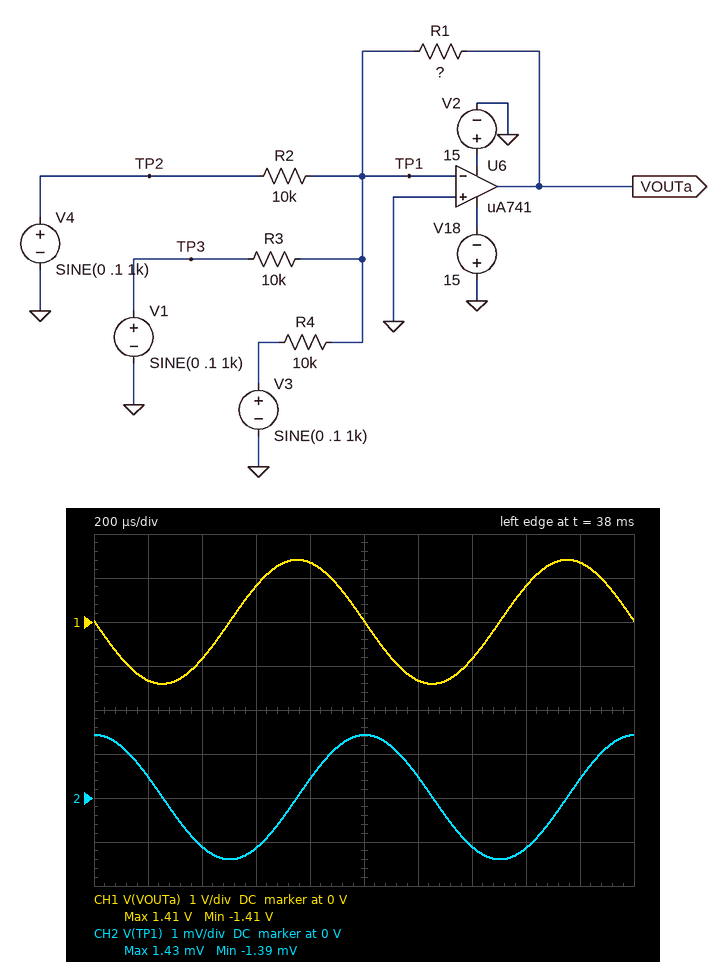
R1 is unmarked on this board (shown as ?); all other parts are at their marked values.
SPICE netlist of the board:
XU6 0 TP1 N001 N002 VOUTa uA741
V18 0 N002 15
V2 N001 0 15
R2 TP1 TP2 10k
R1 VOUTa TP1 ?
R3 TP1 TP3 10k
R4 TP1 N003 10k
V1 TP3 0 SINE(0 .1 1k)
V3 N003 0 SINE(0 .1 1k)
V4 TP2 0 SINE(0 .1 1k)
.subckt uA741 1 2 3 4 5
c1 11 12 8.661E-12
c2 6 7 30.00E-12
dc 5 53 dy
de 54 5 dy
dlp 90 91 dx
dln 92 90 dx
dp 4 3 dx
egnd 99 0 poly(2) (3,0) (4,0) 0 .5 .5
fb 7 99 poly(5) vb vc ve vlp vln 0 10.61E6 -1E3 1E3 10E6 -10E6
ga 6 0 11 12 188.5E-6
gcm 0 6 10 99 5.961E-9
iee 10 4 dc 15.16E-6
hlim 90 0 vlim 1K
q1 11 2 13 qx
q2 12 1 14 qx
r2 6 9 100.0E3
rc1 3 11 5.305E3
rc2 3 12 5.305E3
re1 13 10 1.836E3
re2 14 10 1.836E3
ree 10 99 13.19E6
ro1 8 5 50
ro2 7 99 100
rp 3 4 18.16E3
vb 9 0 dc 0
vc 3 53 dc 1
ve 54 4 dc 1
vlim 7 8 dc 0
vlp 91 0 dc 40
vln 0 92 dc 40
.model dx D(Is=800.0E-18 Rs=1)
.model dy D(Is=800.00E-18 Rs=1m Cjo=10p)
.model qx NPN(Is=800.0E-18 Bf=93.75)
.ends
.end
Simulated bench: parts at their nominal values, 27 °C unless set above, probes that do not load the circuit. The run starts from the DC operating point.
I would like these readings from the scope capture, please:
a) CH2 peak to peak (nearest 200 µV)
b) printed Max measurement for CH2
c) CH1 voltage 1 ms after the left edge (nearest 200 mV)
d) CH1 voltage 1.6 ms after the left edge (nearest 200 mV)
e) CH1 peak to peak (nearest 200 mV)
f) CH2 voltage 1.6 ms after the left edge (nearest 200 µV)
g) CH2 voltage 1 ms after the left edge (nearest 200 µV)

2.8 mV
1.43 mV
0 V
800 mV
2.8 V
-1.2 mV
1.4 mV
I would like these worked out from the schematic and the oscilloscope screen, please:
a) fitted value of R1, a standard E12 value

47 kΩ
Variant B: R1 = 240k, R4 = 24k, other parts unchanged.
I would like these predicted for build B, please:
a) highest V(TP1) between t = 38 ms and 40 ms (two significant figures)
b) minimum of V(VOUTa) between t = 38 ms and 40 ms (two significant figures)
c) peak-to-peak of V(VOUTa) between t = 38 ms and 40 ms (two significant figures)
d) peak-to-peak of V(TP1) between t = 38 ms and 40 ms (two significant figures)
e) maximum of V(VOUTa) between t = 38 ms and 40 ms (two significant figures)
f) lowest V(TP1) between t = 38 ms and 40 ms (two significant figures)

5.8 mV
-5.8 V
12 V
12 mV
5.8 V
-5.8 mV
